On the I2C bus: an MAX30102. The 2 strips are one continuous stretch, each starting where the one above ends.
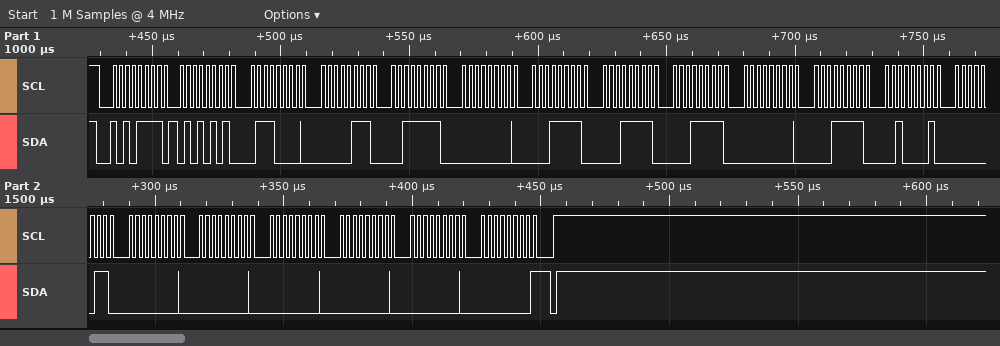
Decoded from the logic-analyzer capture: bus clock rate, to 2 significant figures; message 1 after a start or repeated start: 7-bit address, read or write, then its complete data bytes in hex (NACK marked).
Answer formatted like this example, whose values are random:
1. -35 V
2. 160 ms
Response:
1. 400 kHz
2. 0x57 read: 55 70 07 3F 00 1F 1F 1F 00 1F 21 03 00 00 00 00 00 00 NACK
